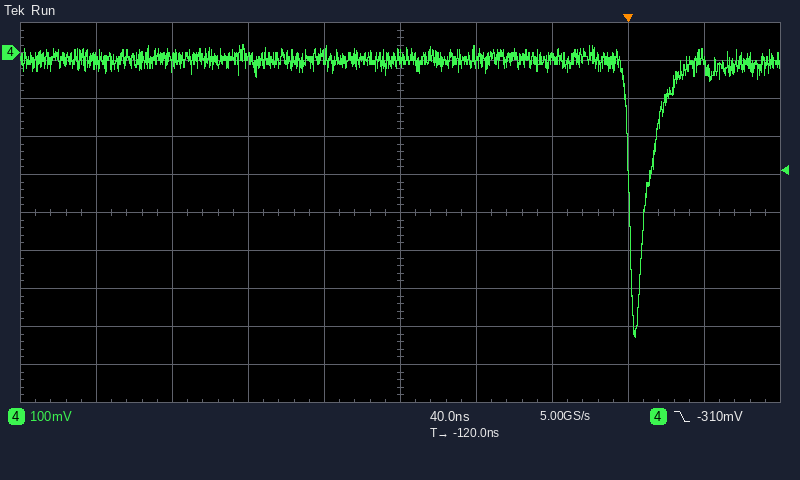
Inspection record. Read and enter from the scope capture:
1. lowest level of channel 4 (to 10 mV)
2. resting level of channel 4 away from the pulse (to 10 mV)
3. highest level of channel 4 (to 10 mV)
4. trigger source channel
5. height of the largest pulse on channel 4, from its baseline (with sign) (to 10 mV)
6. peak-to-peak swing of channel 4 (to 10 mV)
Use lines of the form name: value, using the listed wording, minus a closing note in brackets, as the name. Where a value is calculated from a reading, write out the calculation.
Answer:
lowest level of channel 4: -750 mV
resting level of channel 4 away from the pulse: -20 mV
highest level of channel 4: 20 mV
trigger source channel: channel 4
height of the largest pulse on channel 4, from its baseline (with sign): -750 mV − (-20 mV) = -730 mV
peak-to-peak swing of channel 4: 20 mV − (-750 mV) = 770 mV
